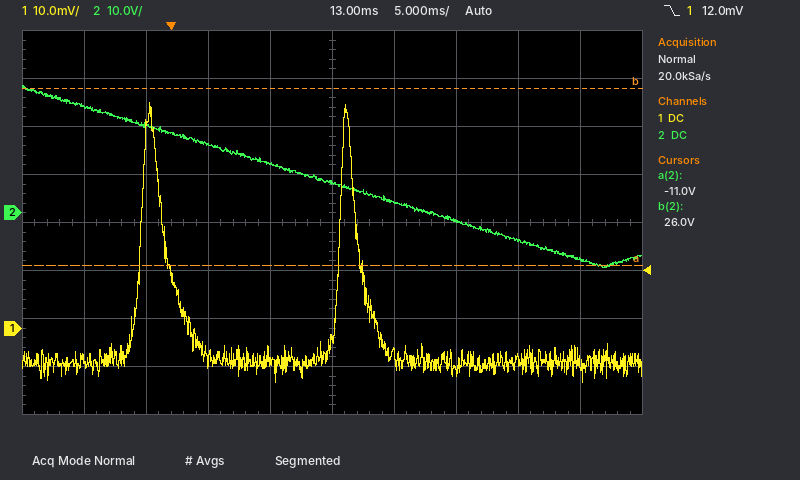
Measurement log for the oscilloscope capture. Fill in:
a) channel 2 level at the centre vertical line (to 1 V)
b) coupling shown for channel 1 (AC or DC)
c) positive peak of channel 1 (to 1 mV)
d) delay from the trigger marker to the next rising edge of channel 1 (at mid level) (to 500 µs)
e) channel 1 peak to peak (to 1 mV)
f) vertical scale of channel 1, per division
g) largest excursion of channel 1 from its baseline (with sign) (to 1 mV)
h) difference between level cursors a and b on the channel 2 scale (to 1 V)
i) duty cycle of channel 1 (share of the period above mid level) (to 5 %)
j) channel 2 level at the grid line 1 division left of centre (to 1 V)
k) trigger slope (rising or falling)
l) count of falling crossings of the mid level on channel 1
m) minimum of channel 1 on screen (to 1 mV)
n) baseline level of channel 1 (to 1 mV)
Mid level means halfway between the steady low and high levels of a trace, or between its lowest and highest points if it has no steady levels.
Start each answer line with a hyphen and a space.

- 6 V
- DC
- 47 mV
- 13.5 ms
- 58 mV
- 10 mV
- +54 mV
- 37 V
- 10 %
- 10 V
- falling
- 2
- -11 mV
- -7 mV
